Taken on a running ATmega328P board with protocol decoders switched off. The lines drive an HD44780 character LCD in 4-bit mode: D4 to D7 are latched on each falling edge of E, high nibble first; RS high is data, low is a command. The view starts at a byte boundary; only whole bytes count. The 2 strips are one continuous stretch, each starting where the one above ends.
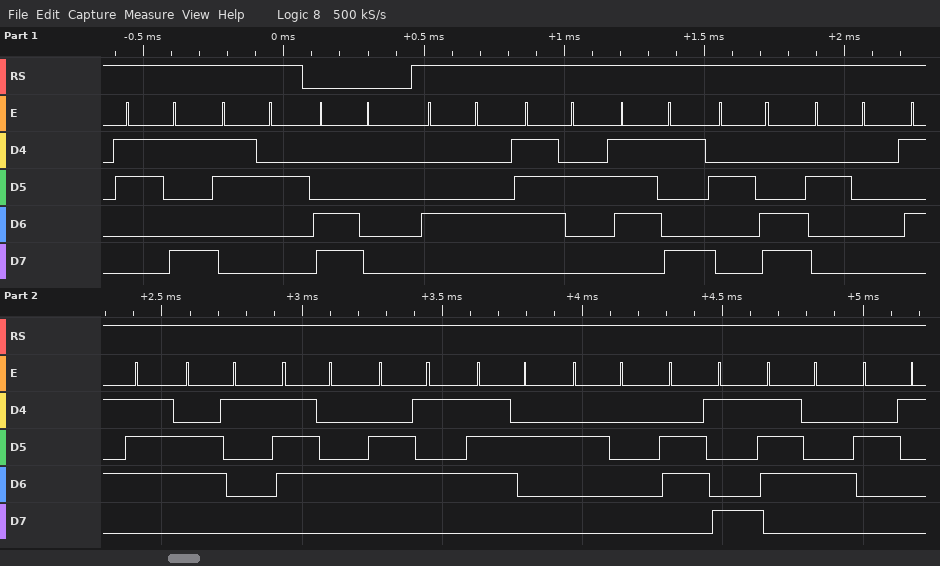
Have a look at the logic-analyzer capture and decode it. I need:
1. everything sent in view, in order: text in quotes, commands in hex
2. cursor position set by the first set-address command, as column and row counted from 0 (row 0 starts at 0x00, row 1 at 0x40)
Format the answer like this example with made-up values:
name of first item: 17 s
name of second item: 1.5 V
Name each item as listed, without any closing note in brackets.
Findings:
everything sent in view, in order: text in quotes, commands in hex: "92" 0xC0 "Dry, Water it!"
cursor position set by the first set-address command, as column and row counted from 0: column 0, row 1
